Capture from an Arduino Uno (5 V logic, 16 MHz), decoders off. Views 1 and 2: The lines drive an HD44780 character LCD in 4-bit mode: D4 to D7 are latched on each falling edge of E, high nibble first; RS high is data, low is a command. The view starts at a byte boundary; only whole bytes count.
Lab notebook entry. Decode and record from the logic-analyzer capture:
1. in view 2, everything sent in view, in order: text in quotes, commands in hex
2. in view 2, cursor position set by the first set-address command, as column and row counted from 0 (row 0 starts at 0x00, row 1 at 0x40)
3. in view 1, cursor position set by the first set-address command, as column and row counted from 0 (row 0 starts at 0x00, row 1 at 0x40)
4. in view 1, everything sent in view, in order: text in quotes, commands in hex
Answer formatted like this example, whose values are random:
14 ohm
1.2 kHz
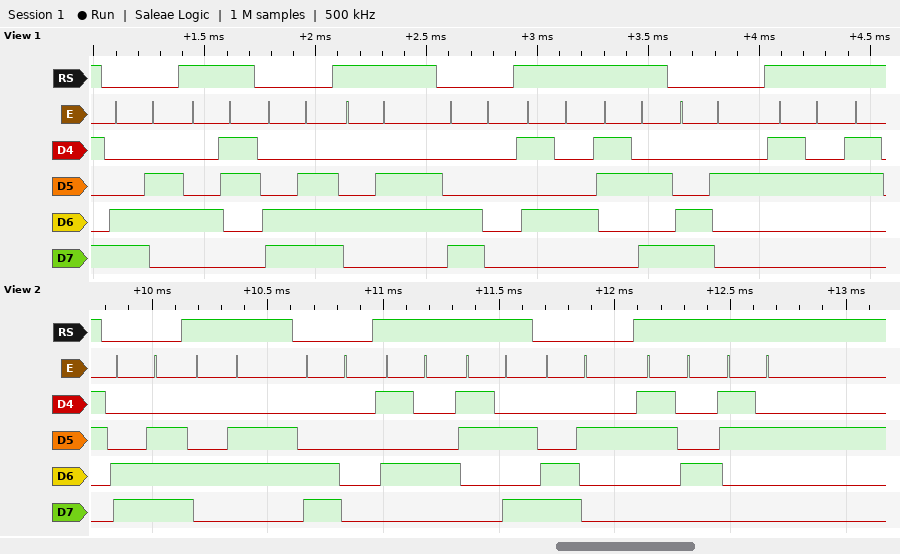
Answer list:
0xCE "F" 0xC0 "T:" 0xC2 "42"
column 14, row 1
column 6, row 1
0xC6 "C" 0xCE "F" 0xC0 "T:" 0xC2 "2"
